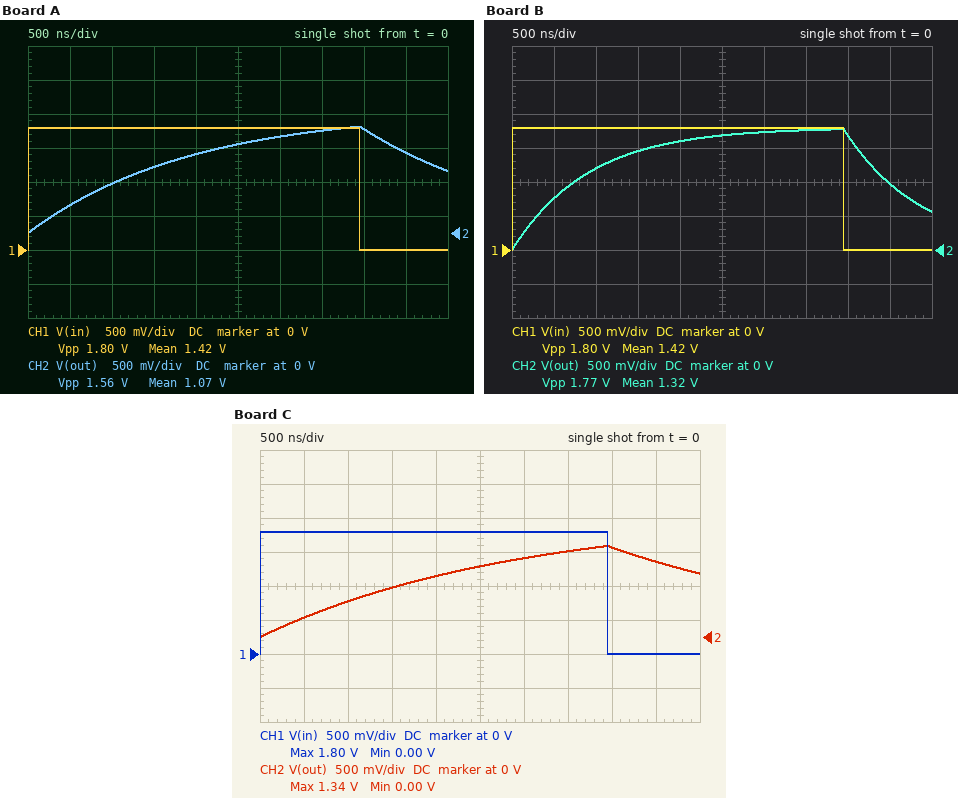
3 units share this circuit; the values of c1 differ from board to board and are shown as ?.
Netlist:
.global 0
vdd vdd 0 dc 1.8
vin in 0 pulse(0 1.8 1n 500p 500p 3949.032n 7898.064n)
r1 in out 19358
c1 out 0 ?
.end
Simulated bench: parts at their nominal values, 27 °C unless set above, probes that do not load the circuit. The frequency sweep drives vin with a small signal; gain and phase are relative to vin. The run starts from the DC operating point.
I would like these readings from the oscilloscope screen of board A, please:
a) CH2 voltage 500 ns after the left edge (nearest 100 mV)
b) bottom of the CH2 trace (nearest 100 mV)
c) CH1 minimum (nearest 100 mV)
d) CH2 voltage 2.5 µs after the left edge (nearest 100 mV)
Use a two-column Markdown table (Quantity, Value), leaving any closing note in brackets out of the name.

| Quantity | Value |
|---|---|
| CH2 voltage 500 ns after the left edge | 400 mV |
| bottom of the CH2 trace | 0 V |
| CH1 minimum | 0 V |
| CH2 voltage 2.5 µs after the left edge | 1.3 V |
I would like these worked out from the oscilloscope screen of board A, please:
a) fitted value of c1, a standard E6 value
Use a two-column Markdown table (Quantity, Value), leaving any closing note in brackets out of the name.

| Quantity | Value |
|---|---|
| fitted value of c1, a standard E6 value | 100 pF |
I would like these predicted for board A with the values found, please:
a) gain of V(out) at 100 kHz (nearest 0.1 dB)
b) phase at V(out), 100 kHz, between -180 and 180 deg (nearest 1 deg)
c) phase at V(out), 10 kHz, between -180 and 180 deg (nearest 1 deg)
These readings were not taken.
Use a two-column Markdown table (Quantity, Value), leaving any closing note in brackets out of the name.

| Quantity | Value |
|---|---|
| gain of V(out) at 100 kHz | -3.9 dB |
| phase at V(out), 100 kHz, between -180 and 180 deg | -51 deg |
| phase at V(out), 10 kHz, between -180 and 180 deg | -7 deg |
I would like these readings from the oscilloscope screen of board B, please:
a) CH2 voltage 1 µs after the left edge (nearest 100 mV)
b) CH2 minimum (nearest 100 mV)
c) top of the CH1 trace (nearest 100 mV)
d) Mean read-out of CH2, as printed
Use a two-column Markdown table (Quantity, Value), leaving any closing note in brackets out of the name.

| Quantity | Value |
|---|---|
| CH2 voltage 1 µs after the left edge | 1.2 V |
| CH2 minimum | 0 V |
| top of the CH1 trace | 1.8 V |
| Mean read-out of CH2, as printed | 1.32 V |
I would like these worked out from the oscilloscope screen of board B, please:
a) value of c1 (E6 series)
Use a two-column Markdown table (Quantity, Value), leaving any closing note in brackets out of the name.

| Quantity | Value |
|---|---|
| value of c1 | 47 pF |
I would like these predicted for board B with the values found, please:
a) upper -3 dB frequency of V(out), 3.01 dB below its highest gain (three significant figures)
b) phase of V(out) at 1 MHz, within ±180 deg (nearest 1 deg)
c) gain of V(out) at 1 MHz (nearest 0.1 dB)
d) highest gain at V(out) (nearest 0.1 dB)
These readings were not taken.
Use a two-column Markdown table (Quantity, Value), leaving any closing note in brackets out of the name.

| Quantity | Value |
|---|---|
| upper -3 dB frequency of V(out), 3.01 dB below its highest gain | 175 kHz |
| phase of V(out) at 1 MHz, within ±180 deg | -80 deg |
| gain of V(out) at 1 MHz | -15.3 dB |
| highest gain at V(out) | 0 dB |
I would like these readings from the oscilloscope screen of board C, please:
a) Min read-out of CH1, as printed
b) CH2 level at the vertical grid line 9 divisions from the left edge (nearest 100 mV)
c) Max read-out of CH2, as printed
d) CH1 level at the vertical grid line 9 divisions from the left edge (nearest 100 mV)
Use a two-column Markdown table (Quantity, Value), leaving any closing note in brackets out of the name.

| Quantity | Value |
|---|---|
| Min read-out of CH1, as printed | 0.00 V |
| CH2 level at the vertical grid line 9 divisions from the left edge | 1.1 V |
| Max read-out of CH2, as printed | 1.34 V |
| CH1 level at the vertical grid line 9 divisions from the left edge | 0 V |
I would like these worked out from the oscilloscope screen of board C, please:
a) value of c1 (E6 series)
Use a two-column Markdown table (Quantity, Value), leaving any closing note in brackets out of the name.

| Quantity | Value |
|---|---|
| value of c1 | 150 pF |
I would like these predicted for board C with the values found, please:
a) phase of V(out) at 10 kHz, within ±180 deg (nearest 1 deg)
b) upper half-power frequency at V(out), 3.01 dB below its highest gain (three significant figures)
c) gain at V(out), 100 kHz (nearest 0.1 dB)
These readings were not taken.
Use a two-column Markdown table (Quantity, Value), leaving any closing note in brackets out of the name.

| Quantity | Value |
|---|---|
| phase of V(out) at 10 kHz, within ±180 deg | -10 deg |
| upper half-power frequency at V(out), 3.01 dB below its highest gain | 54.8 kHz |
| gain at V(out), 100 kHz | -6.4 dB |
